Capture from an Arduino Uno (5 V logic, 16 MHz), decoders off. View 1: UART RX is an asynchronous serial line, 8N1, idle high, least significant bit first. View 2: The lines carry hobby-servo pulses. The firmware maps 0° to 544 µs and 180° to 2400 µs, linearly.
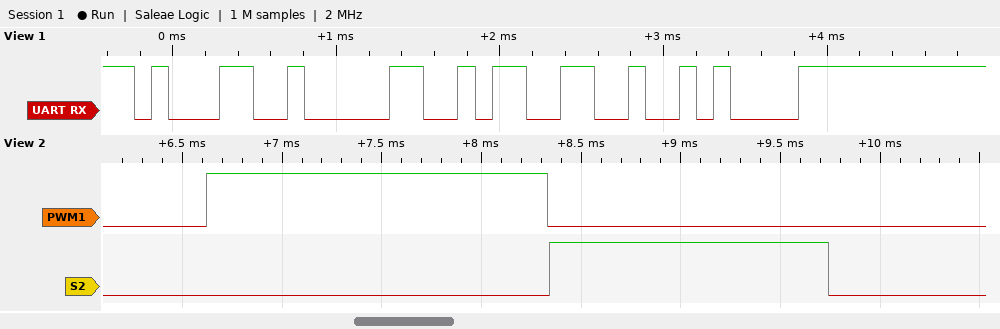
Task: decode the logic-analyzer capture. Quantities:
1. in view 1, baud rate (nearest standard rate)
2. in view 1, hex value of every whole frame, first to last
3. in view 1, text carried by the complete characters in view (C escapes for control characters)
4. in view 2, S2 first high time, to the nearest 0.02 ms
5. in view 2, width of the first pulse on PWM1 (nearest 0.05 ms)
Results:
9600 baud
31 30 33 0A
"103\n"
1.40 ms
1.70 ms
